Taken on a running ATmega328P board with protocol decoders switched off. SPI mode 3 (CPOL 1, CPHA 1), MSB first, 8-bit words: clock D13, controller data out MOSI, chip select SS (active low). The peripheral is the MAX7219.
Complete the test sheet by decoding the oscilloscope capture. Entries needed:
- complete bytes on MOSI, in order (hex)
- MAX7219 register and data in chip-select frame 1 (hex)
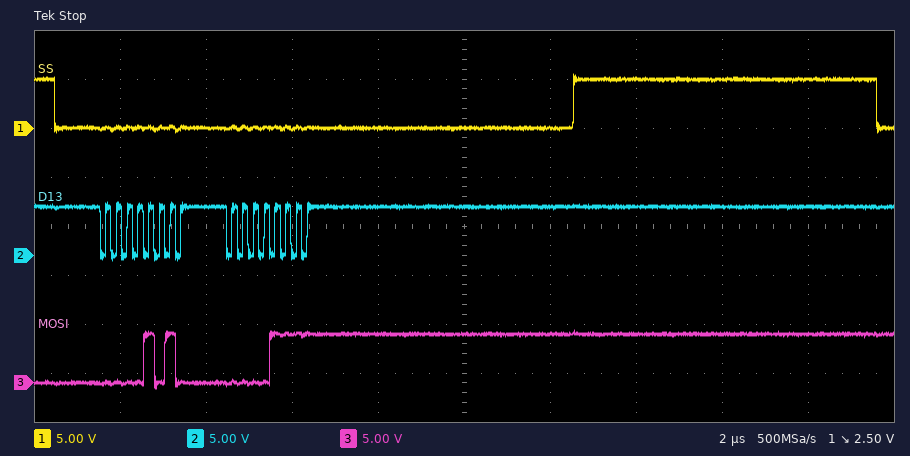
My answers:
0A 0F
register 0xA, data 0x0F
